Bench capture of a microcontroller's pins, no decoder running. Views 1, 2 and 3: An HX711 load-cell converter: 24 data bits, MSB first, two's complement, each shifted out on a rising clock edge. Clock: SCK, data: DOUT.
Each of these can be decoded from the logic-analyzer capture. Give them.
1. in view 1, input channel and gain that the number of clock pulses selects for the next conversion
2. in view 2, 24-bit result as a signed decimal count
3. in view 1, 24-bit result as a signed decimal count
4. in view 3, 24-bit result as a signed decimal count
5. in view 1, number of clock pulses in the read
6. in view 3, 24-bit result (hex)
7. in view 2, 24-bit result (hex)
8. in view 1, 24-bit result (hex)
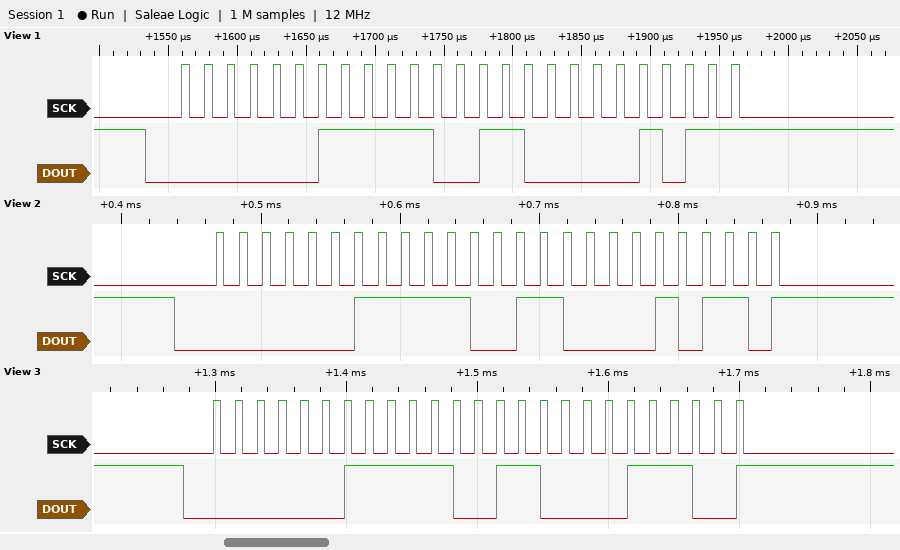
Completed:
channel A, gain 128
255510
255499
255516
25
0x03E61C
0x03E616
0x03E60B
